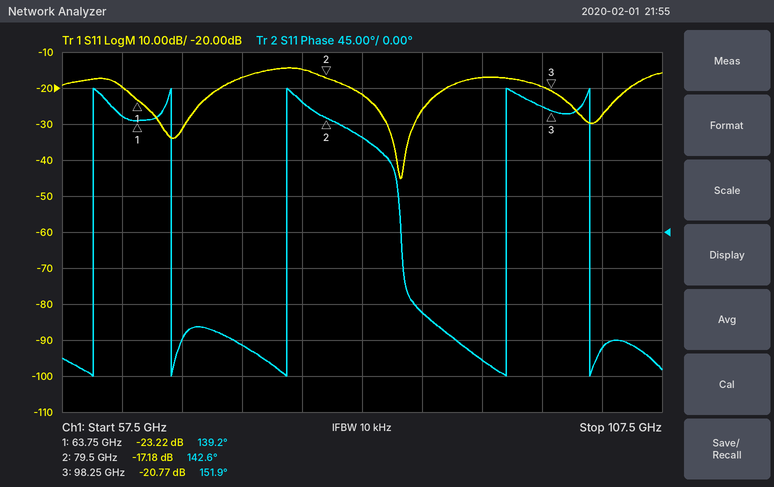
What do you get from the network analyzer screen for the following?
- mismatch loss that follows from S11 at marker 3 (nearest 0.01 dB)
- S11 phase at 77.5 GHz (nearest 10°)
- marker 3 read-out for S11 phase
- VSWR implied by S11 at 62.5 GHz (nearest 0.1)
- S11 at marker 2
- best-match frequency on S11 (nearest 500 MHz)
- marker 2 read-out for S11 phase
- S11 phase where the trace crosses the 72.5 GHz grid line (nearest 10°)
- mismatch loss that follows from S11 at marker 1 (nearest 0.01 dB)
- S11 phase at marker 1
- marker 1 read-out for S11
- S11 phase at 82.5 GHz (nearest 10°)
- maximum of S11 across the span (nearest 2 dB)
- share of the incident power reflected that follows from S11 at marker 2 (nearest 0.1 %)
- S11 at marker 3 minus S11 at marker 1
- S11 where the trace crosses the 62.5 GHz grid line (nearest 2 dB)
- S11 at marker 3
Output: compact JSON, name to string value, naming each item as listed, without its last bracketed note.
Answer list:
{"mismatch loss that follows from S11 at marker 3": "0.04 dB", "S11 phase at 77.5 GHz": "160°", "marker 3 read-out for S11 phase": "151.9°", "VSWR implied by S11 at 62.5 GHz": "1.2", "S11 at marker 2": "-17.18 dB", "best-match frequency on S11": "85.5 GHz", "marker 2 read-out for S11 phase": "142.6°", "S11 phase where the trace crosses the 72.5 GHz grid line": "-140°", "mismatch loss that follows from S11 at marker 1": "0.02 dB", "S11 phase at marker 1": "139.2°", "marker 1 read-out for S11": "-23.22 dB", "S11 phase at 82.5 GHz": "120°", "maximum of S11 across the span": "-14 dB", "share of the incident power reflected that follows from S11 at marker 2": "1.9 %", "S11 at marker 3 minus S11 at marker 1": "2.45 dB", "S11 where the trace crosses the 62.5 GHz grid line": "-20 dB", "S11 at marker 3": "-20.77 dB"}
